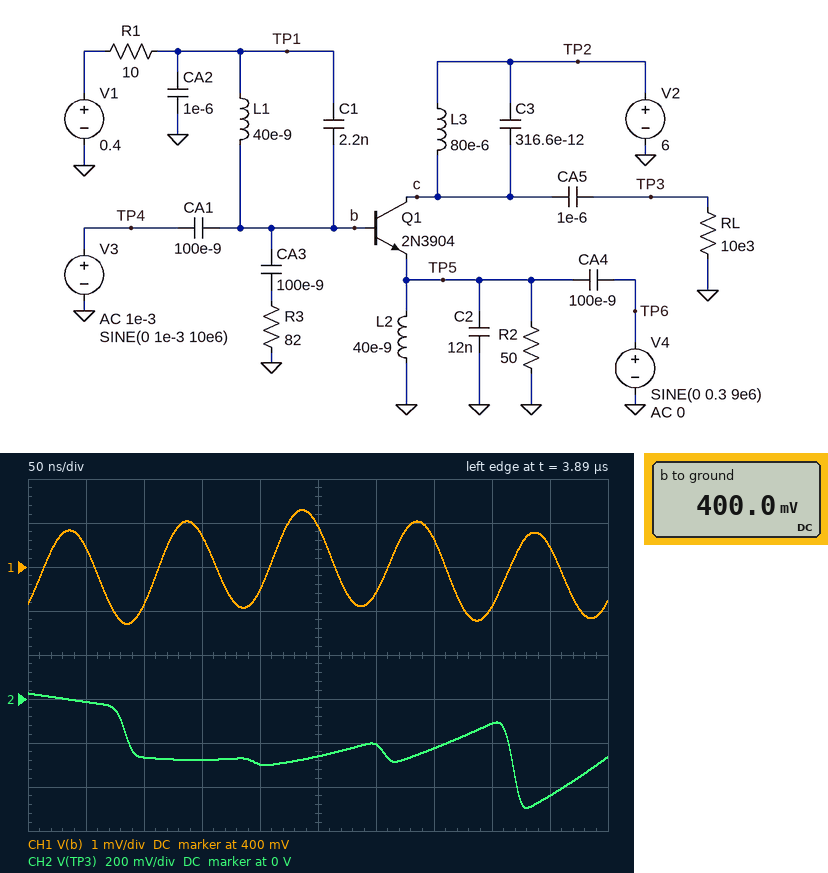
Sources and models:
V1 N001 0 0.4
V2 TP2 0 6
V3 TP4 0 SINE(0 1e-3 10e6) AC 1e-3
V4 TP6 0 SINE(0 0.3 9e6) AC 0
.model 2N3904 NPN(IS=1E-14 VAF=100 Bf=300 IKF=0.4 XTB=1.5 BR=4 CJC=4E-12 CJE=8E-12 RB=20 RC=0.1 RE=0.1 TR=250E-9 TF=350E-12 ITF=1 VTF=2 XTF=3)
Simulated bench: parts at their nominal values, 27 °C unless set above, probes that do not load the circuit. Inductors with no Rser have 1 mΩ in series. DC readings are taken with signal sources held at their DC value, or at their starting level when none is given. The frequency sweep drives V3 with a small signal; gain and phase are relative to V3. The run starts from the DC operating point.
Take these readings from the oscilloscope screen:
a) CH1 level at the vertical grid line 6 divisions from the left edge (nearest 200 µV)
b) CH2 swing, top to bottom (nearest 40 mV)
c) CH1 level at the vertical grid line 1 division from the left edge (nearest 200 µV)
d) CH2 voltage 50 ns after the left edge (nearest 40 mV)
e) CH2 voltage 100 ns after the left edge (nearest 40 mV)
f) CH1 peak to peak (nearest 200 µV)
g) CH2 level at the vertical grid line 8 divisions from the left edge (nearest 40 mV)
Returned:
399.4 mV
520 mV
400.4 mV
0 V
-280 mV
2.6 mV
-120 mV
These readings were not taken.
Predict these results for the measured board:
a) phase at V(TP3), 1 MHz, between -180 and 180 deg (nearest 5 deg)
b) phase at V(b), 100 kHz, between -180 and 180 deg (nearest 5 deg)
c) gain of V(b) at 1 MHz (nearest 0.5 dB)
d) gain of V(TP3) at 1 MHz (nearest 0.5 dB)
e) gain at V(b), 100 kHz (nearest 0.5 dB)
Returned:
-90 deg
10 deg
-24.0 dB
-42.0 dB
-21.0 dB
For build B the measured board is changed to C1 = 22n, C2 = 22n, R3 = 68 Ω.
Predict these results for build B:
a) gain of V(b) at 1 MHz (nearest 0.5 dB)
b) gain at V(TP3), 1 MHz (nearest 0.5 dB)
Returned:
-23.5 dB
-41.5 dB
